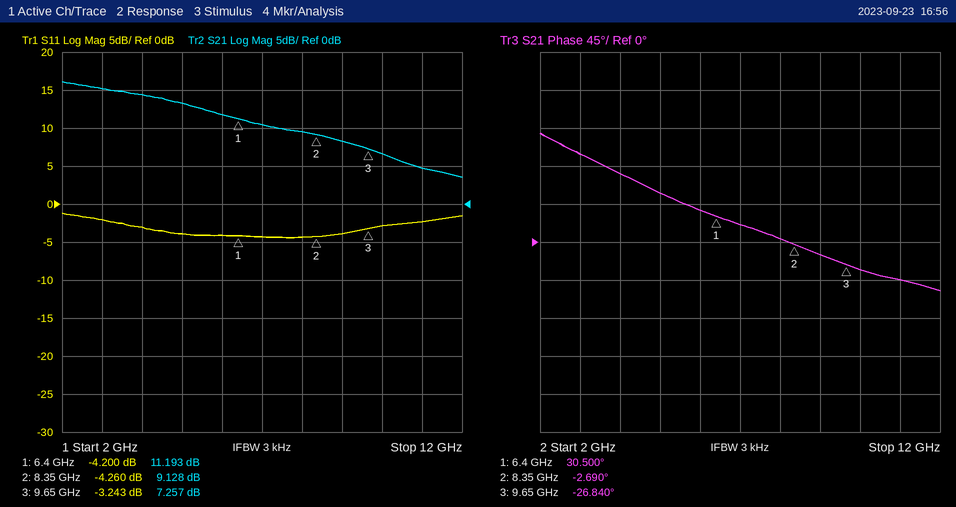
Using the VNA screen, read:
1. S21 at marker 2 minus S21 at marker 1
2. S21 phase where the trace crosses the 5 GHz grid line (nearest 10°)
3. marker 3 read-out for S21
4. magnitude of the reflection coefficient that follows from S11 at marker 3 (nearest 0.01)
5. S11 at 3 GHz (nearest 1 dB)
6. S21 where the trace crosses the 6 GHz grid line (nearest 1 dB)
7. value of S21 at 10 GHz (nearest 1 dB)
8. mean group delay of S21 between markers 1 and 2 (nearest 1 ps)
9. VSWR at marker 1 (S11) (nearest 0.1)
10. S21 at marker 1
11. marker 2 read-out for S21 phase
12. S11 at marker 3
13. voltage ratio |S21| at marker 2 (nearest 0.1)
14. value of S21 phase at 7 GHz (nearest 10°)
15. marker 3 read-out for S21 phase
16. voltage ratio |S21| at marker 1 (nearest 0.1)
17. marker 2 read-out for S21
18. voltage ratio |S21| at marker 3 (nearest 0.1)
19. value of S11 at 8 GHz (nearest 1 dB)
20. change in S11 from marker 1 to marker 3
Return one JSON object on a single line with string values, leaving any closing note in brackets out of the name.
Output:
{"S21 at marker 2 minus S21 at marker 1": "-2.065 dB", "S21 phase where the trace crosses the 5 GHz grid line": "60°", "marker 3 read-out for S21": "7.257 dB", "magnitude of the reflection coefficient that follows from S11 at marker 3": "0.69", "S11 at 3 GHz": "-2 dB", "S21 where the trace crosses the 6 GHz grid line": "12 dB", "value of S21 at 10 GHz": "7 dB", "mean group delay of S21 between markers 1 and 2": "47 ps", "VSWR at marker 1 (S11)": "4.2", "S21 at marker 1": "11.193 dB", "marker 2 read-out for S21 phase": "-2.690°", "S11 at marker 3": "-3.243 dB", "voltage ratio |S21| at marker 2": "2.9", "value of S21 phase at 7 GHz": "20°", "marker 3 read-out for S21 phase": "-26.840°", "voltage ratio |S21| at marker 1": "3.6", "marker 2 read-out for S21": "9.128 dB", "voltage ratio |S21| at marker 3": "2.3", "value of S11 at 8 GHz": "-4 dB", "change in S11 from marker 1 to marker 3": "0.957 dB"}
